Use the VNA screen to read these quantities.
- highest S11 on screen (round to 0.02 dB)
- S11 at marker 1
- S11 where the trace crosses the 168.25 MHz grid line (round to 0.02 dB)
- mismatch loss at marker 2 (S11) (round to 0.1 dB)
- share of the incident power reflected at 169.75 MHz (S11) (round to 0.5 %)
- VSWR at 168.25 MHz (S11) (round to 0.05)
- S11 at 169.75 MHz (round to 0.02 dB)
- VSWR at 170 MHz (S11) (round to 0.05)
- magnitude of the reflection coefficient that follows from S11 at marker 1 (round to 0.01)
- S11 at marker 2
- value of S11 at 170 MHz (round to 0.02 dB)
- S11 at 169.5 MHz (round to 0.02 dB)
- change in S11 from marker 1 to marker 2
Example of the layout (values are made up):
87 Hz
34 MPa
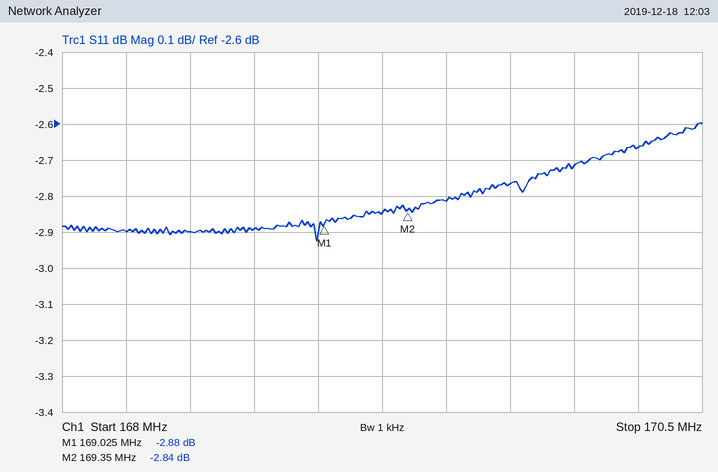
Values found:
-2.60 dB
-2.88 dB
-2.90 dB
3.2 dB
53.0 %
6.05
-2.76 dB
6.45
0.72
-2.84 dB
-2.72 dB
-2.82 dB
0.04 dB
